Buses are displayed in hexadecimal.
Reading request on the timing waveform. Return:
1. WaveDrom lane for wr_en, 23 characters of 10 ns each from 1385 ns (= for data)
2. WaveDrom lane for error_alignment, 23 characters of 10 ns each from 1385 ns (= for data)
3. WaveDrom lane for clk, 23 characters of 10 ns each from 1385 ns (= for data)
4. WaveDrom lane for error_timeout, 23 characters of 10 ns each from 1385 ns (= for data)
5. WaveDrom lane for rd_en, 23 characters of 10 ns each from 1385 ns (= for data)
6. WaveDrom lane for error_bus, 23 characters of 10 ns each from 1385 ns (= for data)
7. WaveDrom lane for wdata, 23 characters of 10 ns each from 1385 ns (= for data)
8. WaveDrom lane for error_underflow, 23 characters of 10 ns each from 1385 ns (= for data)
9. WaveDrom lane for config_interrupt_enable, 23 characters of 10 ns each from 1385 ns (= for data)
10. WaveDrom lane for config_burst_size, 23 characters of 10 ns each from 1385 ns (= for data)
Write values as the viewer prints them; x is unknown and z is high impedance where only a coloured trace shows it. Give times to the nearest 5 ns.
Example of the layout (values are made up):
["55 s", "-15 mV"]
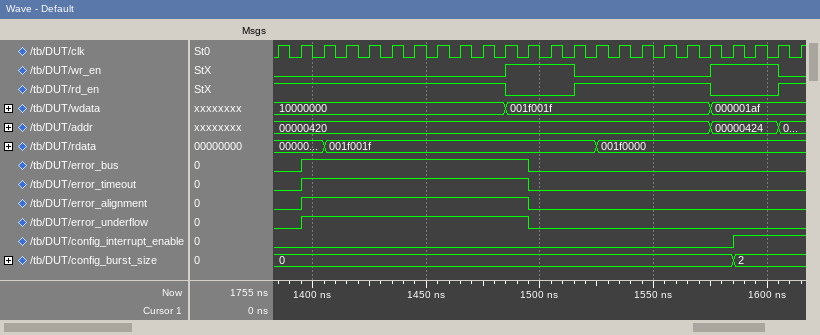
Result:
["{name: 'wr_en', wave: '0.........1..0.....1..0'}", "{name: 'error_alignment', wave: '01.........0...........'}", "{name: 'clk', wave: 'p......................'}", "{name: 'error_timeout', wave: '01.........0...........'}", "{name: 'rd_en', wave: '1.........0..1.....0..1'}", "{name: 'error_bus', wave: '01.........0...........'}", "{name: 'wdata', wave: '=.........=........=...', data: '10000000 001f001f 000001af'}", "{name: 'error_underflow', wave: '01.........0...........'}", "{name: 'config_interrupt_enable', wave: '0...................1..'}", "{name: 'config_burst_size', wave: '=...................=..', data: '0 2'}"]
